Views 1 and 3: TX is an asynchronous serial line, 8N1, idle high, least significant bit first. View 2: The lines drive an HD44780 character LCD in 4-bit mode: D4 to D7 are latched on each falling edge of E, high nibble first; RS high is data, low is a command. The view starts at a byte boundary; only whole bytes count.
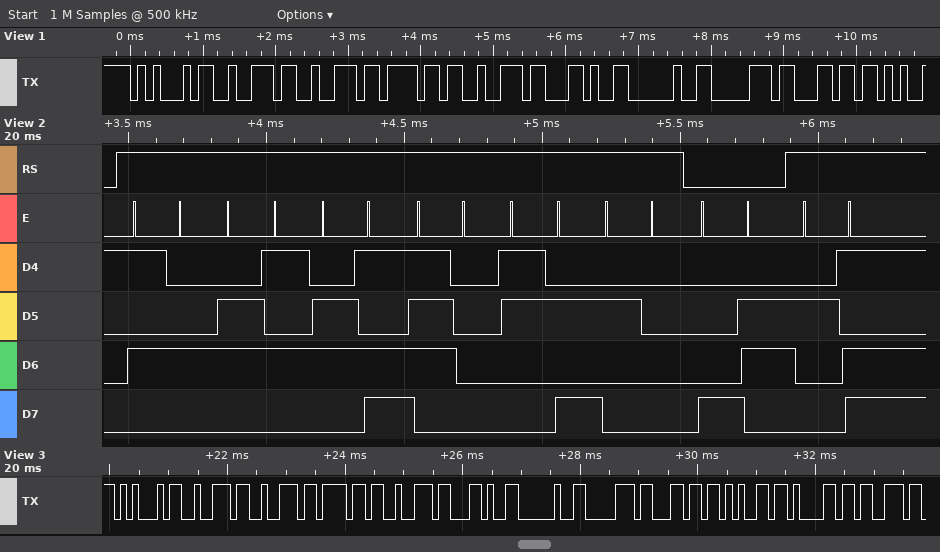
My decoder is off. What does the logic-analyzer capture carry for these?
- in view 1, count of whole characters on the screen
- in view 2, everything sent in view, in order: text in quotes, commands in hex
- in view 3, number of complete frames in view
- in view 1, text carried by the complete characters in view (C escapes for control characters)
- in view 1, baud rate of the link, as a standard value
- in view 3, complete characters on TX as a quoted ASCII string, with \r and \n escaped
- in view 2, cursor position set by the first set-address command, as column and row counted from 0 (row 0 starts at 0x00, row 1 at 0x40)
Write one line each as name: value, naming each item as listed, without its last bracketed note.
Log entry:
in view 1, count of whole characters on the screen: 9
in view 2, everything sent in view, in order: text in quotes, commands in hex: "Temp: " 0x86 "-"
in view 3, number of complete frames in view: 12
in view 1, text carried by the complete characters in view: "Error, pl"
in view 1, baud rate of the link, as a standard value: 9600 baud
in view 3, complete characters on TX as a quoted ASCII string, with \r and \n escaped: "Error, pleas"
in view 2, cursor position set by the first set-address command, as column and row counted from 0: column 6, row 0
